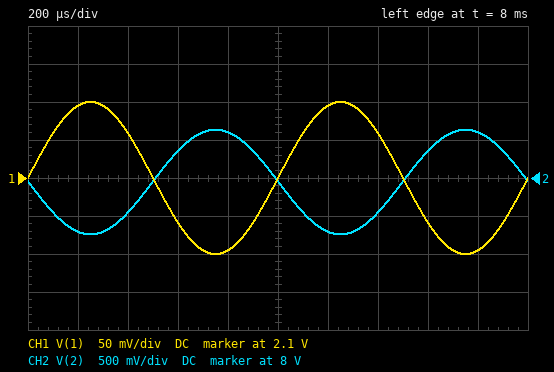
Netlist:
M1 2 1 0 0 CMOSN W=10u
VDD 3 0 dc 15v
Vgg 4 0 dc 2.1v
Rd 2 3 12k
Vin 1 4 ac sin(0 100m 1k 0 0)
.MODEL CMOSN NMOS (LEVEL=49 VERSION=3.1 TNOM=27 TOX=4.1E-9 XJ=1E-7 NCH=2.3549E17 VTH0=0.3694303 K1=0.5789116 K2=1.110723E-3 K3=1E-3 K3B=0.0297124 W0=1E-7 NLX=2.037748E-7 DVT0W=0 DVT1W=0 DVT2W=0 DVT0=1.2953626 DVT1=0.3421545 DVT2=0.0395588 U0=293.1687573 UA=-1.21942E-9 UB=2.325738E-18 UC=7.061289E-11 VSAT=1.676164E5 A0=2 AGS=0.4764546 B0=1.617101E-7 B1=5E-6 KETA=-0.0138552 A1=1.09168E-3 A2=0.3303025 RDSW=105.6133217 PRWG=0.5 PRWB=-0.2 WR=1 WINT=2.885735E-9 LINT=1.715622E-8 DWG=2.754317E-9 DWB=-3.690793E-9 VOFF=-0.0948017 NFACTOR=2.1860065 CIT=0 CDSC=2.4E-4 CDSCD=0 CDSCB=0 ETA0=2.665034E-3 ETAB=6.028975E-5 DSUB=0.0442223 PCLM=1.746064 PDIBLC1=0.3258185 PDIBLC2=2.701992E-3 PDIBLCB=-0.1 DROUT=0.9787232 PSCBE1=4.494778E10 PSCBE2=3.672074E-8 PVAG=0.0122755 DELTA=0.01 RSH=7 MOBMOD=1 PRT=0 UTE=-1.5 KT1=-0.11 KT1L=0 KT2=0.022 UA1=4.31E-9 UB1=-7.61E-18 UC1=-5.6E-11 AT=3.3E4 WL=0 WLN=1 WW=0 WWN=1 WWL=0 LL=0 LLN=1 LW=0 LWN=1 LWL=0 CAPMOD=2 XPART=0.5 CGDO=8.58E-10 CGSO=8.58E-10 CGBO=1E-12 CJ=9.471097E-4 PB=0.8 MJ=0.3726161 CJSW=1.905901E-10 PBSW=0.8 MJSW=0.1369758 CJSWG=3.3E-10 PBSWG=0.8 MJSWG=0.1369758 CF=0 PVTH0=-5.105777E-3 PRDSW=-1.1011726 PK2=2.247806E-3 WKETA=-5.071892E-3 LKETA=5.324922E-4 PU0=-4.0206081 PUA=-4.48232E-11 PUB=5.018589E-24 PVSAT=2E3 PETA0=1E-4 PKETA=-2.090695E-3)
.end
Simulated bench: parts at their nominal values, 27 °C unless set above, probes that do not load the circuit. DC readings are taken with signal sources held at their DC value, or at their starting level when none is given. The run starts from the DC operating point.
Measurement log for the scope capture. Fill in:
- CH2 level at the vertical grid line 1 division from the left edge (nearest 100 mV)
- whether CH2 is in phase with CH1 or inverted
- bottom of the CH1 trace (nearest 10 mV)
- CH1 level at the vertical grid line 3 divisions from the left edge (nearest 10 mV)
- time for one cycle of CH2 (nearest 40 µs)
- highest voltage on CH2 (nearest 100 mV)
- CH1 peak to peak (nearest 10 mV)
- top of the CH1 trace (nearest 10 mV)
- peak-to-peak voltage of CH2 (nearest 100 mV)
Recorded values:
7.3 V
inverted
2.00 V
2.04 V
1.00 ms
8.6 V
200 mV
2.20 V
1.4 V
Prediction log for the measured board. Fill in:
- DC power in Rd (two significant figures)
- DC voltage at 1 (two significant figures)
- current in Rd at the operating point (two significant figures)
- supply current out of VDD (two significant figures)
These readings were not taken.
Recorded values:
4.1 mW
2.1 V
590 µA
590 µA
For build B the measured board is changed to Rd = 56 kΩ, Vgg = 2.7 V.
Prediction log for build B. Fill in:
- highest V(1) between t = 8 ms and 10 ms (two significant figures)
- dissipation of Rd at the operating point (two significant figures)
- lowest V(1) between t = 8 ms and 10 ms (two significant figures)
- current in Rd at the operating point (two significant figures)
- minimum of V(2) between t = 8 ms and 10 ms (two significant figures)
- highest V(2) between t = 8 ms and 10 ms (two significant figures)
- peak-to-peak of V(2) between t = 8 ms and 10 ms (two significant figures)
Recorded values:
2.8 V
3.8 mW
2.6 V
260 µA
350 mV
360 mV
6.6 mV
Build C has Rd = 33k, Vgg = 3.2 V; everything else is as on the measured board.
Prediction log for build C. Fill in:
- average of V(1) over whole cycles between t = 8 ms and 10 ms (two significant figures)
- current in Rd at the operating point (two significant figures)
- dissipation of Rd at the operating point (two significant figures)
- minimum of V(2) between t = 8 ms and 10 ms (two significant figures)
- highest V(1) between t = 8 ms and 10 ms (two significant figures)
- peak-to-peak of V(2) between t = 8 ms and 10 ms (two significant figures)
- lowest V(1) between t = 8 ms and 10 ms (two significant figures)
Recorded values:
3.2 V
440 µA
6.3 mW
610 mV
3.3 V
1.9 mV
3.1 V
